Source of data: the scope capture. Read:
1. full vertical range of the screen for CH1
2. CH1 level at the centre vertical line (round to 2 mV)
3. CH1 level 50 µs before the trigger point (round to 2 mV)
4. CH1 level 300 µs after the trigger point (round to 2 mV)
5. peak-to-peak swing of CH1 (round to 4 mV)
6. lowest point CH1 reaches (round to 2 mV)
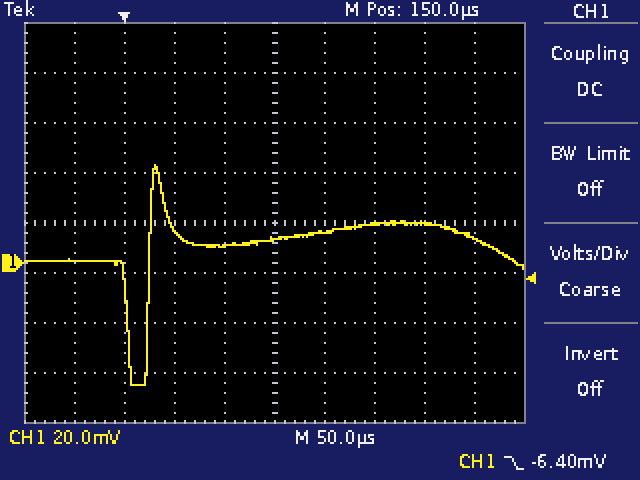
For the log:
160 mV
10 mV
0 mV
16 mV
88 mV
-48 mV
